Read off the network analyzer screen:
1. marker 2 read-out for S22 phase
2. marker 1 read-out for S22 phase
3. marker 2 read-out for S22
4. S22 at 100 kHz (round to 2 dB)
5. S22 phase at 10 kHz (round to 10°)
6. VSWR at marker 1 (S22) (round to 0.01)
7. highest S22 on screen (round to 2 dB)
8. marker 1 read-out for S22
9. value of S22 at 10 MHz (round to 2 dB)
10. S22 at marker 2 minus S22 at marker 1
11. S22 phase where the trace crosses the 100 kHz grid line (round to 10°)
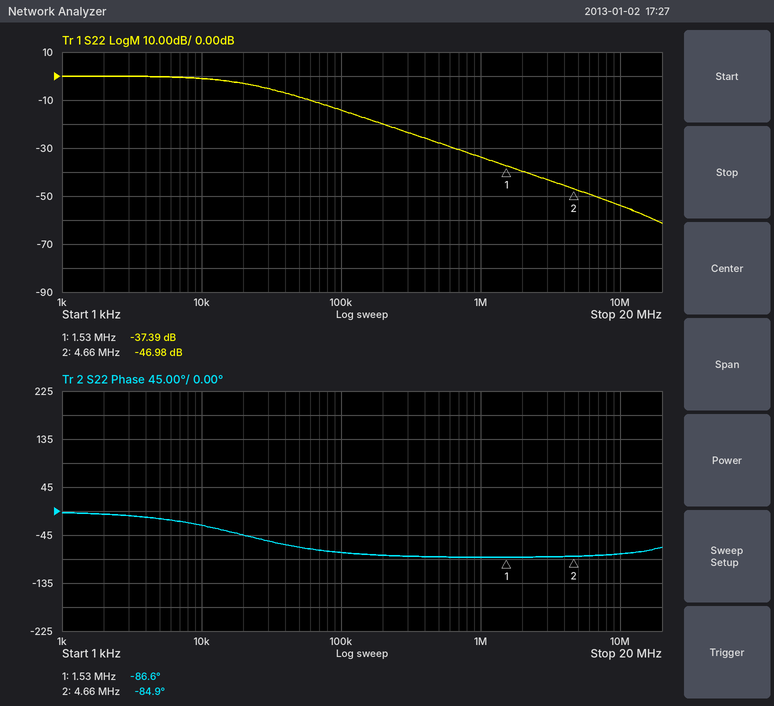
-84.9°
-86.6°
-46.98 dB
-14 dB
-30°
1.03
0 dB
-37.39 dB
-54 dB
-9.59 dB
-80°
